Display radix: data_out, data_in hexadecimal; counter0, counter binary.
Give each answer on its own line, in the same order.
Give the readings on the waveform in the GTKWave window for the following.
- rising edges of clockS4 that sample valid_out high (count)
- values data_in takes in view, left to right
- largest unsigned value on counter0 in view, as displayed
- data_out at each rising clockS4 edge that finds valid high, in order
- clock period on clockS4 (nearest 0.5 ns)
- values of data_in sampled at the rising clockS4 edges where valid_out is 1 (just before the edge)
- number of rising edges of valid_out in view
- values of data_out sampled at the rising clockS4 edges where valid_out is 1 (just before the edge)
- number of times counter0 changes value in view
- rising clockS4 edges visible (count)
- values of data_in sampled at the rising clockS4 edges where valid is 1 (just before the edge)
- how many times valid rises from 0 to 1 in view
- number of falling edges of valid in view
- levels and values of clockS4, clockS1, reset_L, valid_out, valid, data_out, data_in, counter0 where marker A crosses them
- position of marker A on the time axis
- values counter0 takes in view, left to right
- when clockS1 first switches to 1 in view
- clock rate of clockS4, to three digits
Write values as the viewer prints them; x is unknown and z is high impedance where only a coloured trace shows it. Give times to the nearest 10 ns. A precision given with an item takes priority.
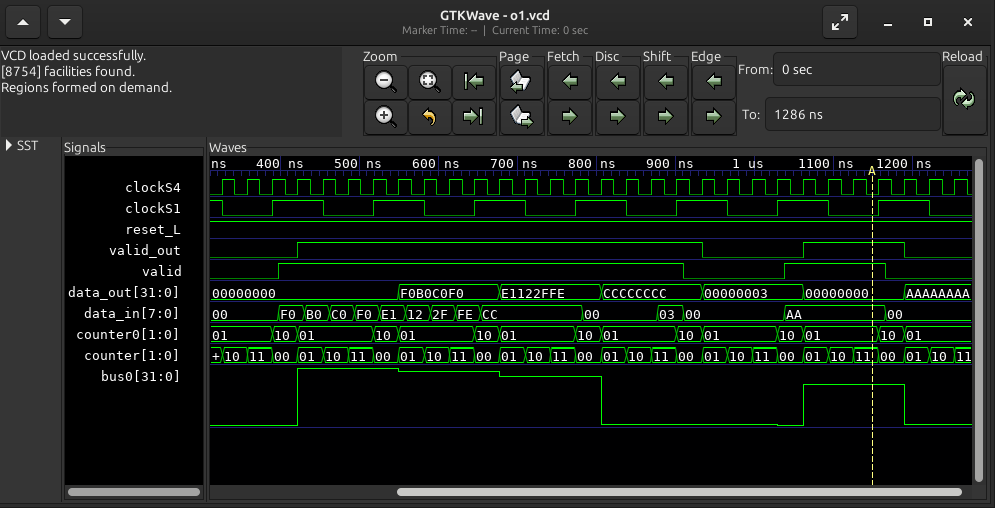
20
00, F0, B0, C0, F0, E1, 12, 2F, FE, CC, 00, 03, 00, AA, 00
10
00000000, 00000000, 00000000, 00000000, 00000000, F0B0C0F0, F0B0C0F0, F0B0C0F0, F0B0C0F0, E1122FFE, E1122FFE, E1122FFE, E1122FFE, CCCCCCCC, CCCCCCCC, CCCCCCCC, 00000003, 00000000, 00000000, 00000000
32 ns
B0, C0, F0, E1, 12, 2F, FE, CC, CC, CC, CC, 00, 00, 00, 03, 00, AA, AA, AA, 00
2
00000000, 00000000, 00000000, 00000000, F0B0C0F0, F0B0C0F0, F0B0C0F0, F0B0C0F0, E1122FFE, E1122FFE, E1122FFE, E1122FFE, CCCCCCCC, CCCCCCCC, CCCCCCCC, CCCCCCCC, 00000000, 00000000, 00000000, 00000000
14
30
F0, B0, C0, F0, E1, 12, 2F, FE, CC, CC, CC, CC, 00, 00, 00, 03, AA, AA, AA, AA
2
2
clockS4=0, clockS1=0, reset_L=1, valid_out=1, valid=1, data_out=00000000, data_in=AA, counter0=01
1150 ns
01, 10, 01, 10, 01, 10, 01, 10, 01, 10, 01, 10, 01, 10, 01
390 ns
31.2 MHz
